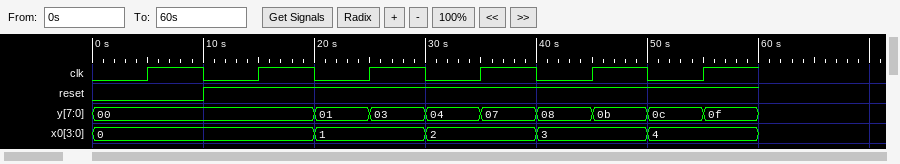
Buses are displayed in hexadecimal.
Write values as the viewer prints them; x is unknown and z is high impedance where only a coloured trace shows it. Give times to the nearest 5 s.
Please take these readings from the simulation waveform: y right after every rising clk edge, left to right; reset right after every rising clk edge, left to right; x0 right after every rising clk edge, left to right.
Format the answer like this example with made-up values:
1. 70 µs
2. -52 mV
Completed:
1. 00, 00, 03, 07, 0b, 0f
2. 0 1 1 1 1 1
3. 0, 0, 1, 2, 3, 4
